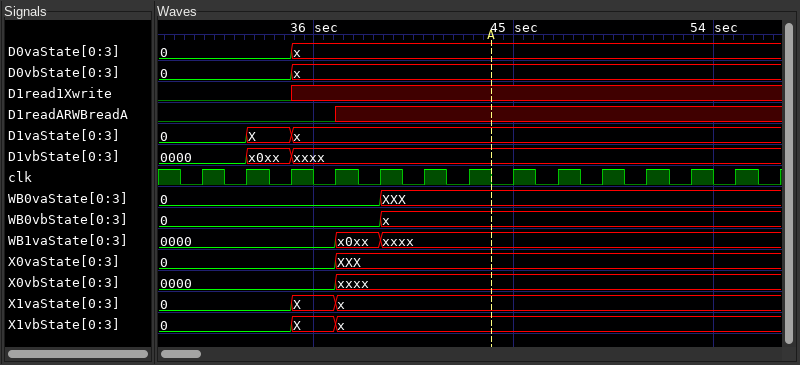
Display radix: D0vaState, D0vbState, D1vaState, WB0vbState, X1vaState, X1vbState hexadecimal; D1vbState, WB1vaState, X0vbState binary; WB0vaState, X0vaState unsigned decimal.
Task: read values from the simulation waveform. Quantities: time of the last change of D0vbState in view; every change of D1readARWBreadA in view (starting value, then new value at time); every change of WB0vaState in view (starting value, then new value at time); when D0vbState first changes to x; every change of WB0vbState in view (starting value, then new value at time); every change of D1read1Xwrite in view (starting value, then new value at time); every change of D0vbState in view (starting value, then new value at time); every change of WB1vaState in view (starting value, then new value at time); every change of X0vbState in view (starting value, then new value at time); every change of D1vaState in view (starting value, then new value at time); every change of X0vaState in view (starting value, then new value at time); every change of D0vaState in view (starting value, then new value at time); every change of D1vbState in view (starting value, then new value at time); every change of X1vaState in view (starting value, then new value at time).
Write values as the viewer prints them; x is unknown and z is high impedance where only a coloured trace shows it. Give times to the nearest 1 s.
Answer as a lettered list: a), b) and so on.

a) 35 s
b) 0, x at 37 s
c) 0, XXX at 39 s
d) 35 s
e) 0, x at 39 s
f) 0, x at 35 s
g) 0, x at 35 s
h) 0000, x0xx at 37 s, xxxx at 39 s
i) 0000, xxxx at 37 s
j) 0, X at 33 s, x at 35 s
k) 0, XXX at 37 s
l) 0, x at 35 s
m) 0000, x0xx at 33 s, xxxx at 35 s
n) 0, X at 35 s, x at 37 s
